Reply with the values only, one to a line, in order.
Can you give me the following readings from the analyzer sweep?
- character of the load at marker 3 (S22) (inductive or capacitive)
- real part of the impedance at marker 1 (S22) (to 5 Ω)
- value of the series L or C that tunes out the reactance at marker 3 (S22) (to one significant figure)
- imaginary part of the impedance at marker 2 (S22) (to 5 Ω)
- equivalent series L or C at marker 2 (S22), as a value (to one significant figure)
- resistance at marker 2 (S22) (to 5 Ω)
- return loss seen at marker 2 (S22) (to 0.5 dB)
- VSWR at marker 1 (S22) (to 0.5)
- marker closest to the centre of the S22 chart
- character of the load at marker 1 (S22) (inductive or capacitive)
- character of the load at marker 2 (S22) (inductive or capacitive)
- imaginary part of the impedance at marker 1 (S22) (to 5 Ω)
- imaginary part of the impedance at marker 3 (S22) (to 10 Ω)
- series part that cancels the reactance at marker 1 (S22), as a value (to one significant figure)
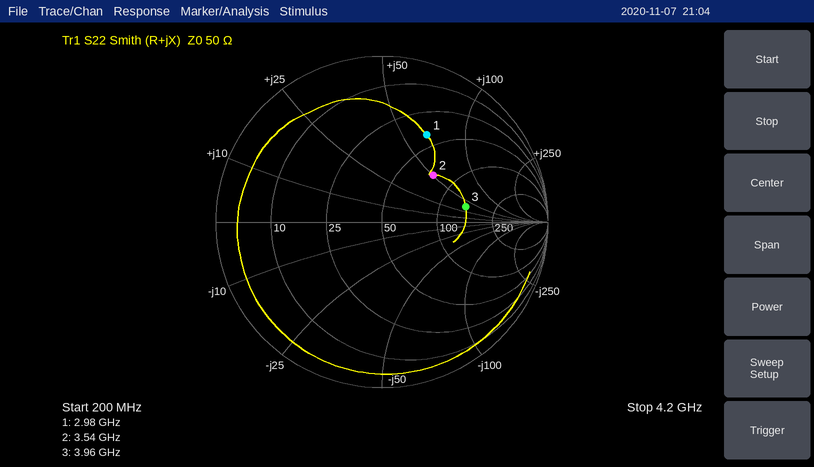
inductive
40 Ω
1 pF
+50 Ω
2 nH
75 Ω
7.5 dB
4.0
marker 2
inductive
inductive
+65 Ω
+40 Ω
800 fF
